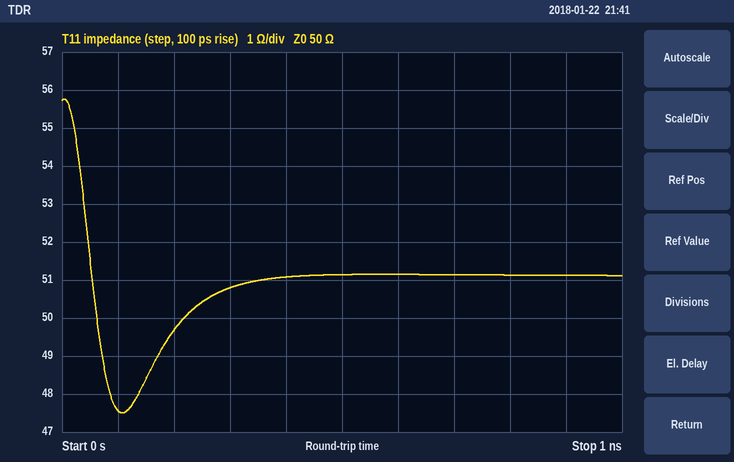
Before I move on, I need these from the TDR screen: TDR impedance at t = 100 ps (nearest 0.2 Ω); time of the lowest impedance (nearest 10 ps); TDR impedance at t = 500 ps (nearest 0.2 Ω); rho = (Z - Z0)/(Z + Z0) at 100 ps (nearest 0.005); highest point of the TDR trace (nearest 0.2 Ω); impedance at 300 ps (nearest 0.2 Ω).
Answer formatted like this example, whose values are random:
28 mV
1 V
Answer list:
47.6 Ω
110 ps
51.2 Ω
-0.025
55.8 Ω
50.8 Ω
